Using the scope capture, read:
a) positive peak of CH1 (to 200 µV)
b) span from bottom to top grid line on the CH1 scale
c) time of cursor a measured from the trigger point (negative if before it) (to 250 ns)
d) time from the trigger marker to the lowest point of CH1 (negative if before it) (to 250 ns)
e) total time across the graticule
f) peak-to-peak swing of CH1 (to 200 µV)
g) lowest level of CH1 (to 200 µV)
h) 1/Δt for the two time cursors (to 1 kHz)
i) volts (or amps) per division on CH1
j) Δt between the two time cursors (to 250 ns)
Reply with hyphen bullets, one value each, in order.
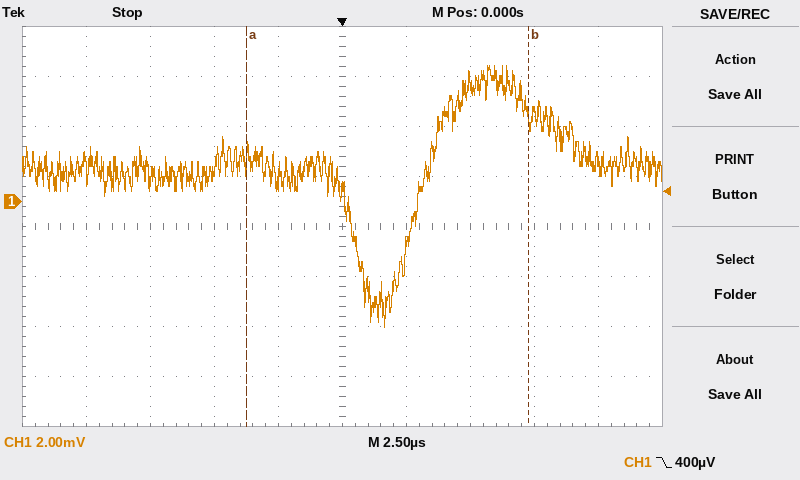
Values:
- 5.4 mV
- 16 mV
- -3.75 µs
- +1.75 µs
- 25 µs
- 10.4 mV
- -5.0 mV
- 91 kHz
- 2 mV
- 11.00 µs
